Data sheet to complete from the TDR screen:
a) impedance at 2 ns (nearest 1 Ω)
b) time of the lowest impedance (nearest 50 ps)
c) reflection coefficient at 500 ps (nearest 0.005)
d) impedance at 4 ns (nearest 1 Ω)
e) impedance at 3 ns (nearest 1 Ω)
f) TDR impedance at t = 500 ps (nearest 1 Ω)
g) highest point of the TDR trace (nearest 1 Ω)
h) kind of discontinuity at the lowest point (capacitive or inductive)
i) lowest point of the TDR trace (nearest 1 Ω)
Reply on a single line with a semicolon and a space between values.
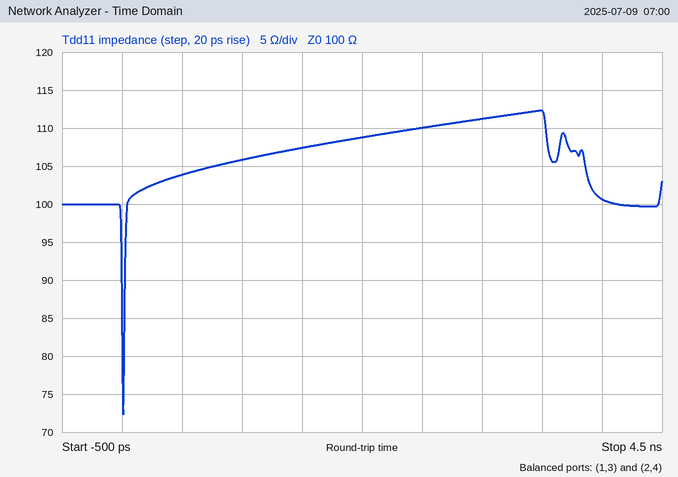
109 Ω; 0 ps; +0.020; 101 Ω; 111 Ω; 104 Ω; 112 Ω; capacitive; 72 Ω
